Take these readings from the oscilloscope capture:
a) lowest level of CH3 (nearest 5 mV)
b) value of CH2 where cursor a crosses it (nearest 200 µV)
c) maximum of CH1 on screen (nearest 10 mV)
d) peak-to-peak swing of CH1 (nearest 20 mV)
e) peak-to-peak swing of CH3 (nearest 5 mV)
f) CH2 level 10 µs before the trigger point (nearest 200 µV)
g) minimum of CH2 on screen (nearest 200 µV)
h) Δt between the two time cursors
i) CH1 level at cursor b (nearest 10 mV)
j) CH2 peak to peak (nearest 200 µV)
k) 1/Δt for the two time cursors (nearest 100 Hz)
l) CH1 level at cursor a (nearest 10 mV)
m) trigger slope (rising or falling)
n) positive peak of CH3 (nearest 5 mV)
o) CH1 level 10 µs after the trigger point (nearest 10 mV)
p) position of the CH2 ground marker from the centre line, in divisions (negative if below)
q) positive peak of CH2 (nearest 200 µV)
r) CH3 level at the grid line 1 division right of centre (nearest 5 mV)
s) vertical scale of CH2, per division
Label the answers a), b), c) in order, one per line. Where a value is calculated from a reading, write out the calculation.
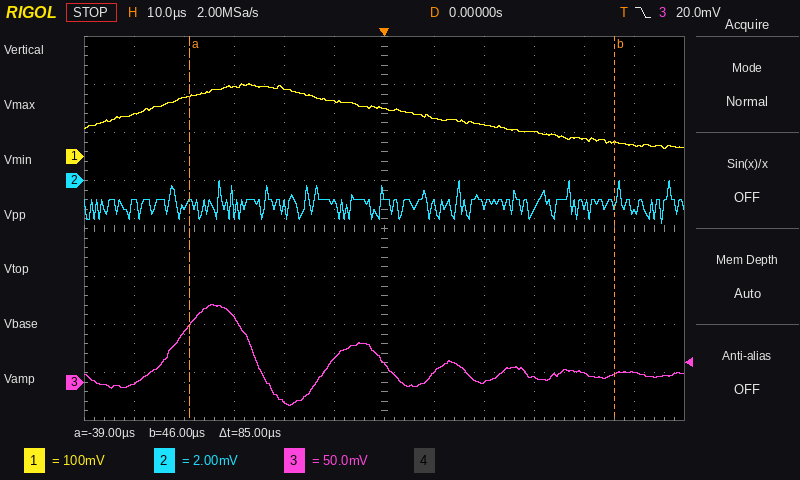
a) -25 mV
b) -1.0 mV
c) 150 mV
d) 140 mV
e) 80 mV − (-25 mV) = 105 mV
f) -1.0 mV
g) -1.8 mV
h) 85 µs
i) 30 mV
j) 0.0 mV − (-1.8 mV) = 1.8 mV
k) 1 / 85 µs ≈ 11.8 kHz
l) 130 mV
m) falling
n) 80 mV
o) 80 mV
p) +1.0 div
q) 0.0 mV
r) 10 mV
s) 2 mV
